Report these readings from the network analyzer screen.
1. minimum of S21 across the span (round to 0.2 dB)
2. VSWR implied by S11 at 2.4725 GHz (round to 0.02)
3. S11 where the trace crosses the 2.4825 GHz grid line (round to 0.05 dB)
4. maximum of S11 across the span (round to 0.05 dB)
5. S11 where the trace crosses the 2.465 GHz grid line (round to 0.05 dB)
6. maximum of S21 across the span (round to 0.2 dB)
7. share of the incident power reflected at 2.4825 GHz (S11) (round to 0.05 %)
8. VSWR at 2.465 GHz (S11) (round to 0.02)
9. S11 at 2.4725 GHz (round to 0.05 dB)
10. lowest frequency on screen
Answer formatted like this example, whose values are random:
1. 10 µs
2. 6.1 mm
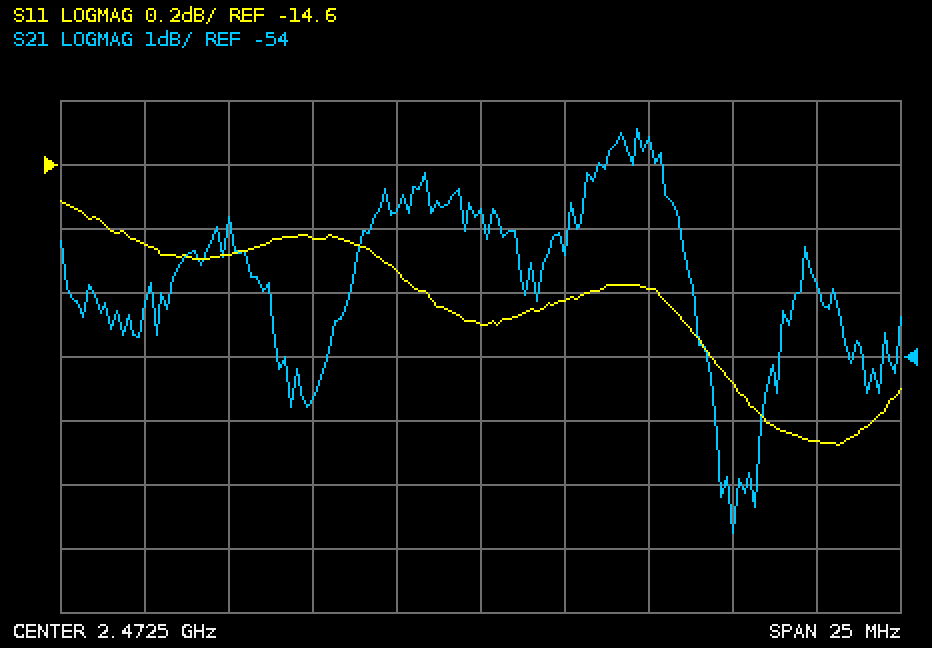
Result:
1. -56.8 dB
2. 1.42
3. -15.45 dB
4. -14.70 dB
5. -14.90 dB
6. -50.4 dB
7. 2.85 %
8. 1.44
9. -15.10 dB
10. 2.46 GHz
